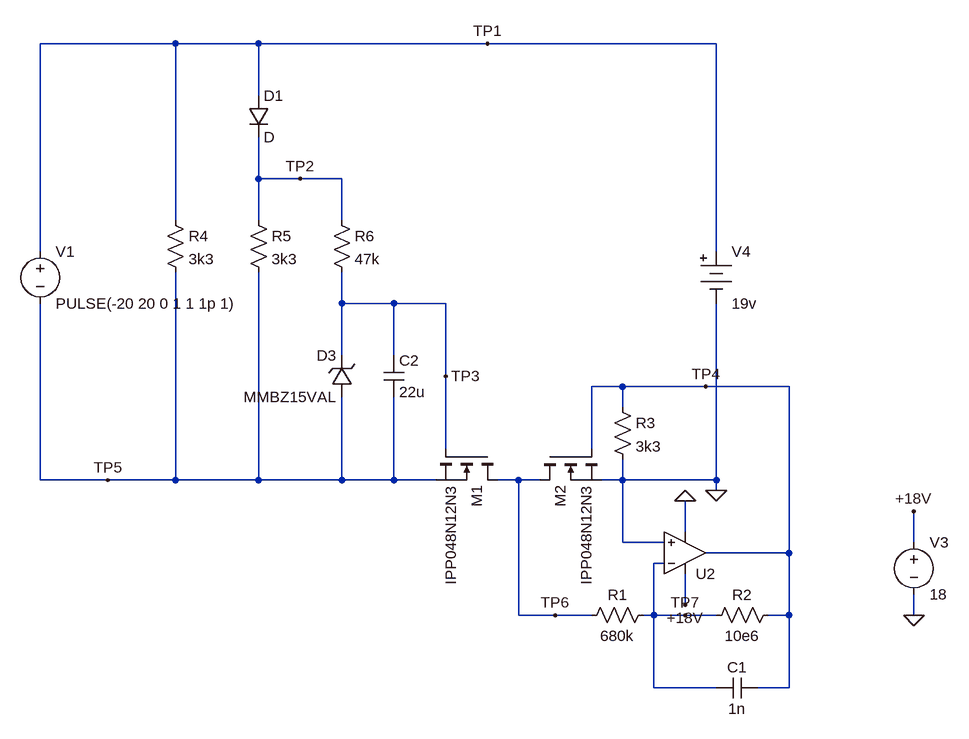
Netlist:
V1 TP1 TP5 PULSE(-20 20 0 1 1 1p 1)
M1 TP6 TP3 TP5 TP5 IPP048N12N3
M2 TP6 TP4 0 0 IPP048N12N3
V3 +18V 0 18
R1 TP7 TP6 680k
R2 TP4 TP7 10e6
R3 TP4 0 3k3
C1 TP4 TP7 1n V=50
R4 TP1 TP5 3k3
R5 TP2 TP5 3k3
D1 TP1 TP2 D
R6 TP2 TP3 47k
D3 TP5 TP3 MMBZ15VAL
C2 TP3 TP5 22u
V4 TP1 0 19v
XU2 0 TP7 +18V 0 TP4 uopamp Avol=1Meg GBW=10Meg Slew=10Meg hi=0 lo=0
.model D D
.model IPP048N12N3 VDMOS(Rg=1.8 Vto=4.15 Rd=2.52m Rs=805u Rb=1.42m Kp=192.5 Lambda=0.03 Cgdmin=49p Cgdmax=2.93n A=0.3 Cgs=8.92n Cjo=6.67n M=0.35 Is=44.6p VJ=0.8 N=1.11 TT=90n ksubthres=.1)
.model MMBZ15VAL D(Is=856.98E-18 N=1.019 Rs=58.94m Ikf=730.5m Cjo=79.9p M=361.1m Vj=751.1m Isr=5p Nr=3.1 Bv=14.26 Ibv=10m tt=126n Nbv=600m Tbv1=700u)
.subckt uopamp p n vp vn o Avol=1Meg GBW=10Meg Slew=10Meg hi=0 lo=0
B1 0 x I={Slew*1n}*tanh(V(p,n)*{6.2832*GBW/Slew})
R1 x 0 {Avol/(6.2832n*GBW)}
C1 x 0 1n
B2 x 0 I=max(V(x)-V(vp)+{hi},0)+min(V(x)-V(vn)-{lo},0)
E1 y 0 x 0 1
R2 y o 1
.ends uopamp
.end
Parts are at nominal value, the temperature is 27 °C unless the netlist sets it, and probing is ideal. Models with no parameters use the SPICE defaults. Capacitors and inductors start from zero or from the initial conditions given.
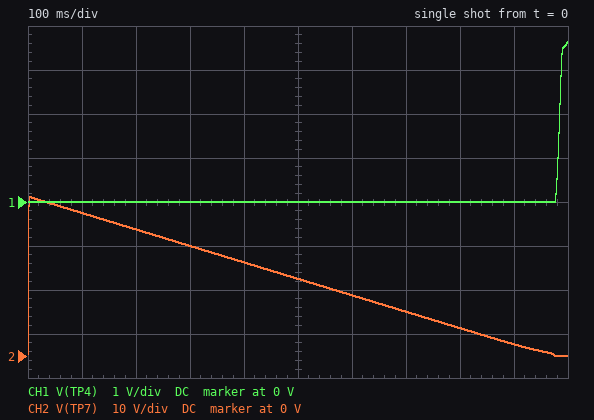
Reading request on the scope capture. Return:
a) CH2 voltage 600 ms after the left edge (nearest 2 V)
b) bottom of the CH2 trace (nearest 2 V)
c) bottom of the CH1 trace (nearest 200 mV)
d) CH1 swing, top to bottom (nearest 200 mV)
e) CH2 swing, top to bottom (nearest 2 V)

14 V
0 V
0 V
3.6 V
36 V
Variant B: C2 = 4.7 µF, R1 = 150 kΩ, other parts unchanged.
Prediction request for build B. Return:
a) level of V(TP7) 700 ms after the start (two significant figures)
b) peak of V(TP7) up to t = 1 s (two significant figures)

11 V
38 V
